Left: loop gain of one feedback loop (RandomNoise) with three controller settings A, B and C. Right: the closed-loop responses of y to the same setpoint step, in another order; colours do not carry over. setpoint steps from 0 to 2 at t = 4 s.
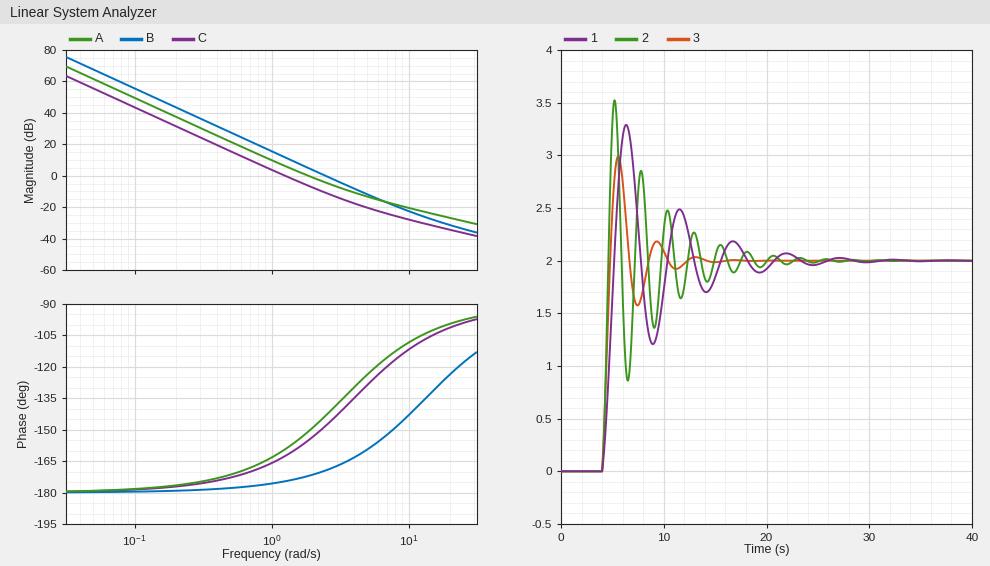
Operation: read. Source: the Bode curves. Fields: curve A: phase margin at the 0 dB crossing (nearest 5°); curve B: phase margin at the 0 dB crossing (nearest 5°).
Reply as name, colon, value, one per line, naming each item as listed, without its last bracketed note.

curve A: phase margin at the 0 dB crossing: 30°
curve B: phase margin at the 0 dB crossing: 10°
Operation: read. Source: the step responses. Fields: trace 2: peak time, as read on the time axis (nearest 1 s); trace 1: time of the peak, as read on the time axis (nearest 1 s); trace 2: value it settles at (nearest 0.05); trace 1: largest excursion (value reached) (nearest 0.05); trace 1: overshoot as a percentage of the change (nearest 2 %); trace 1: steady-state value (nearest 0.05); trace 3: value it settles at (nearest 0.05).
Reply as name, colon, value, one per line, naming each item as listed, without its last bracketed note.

trace 2: peak time, as read on the time axis: 5 s
trace 1: time of the peak, as read on the time axis: 6 s
trace 2: value it settles at: 2.00
trace 1: largest excursion (value reached): 3.30
trace 1: overshoot as a percentage of the change: 64 %
trace 1: steady-state value: 2.00
trace 3: value it settles at: 2.00
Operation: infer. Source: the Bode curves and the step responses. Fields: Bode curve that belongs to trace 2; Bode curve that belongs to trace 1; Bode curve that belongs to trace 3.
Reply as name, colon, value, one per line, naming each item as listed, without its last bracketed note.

Bode curve that belongs to trace 2: B
Bode curve that belongs to trace 1: C
Bode curve that belongs to trace 3: A
